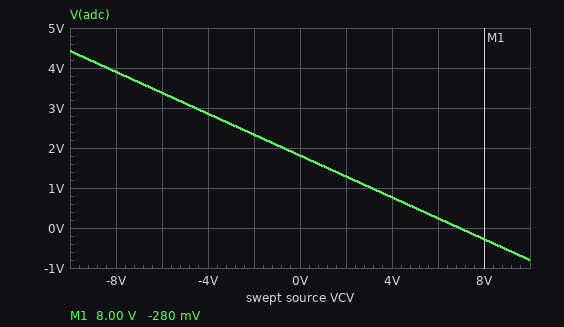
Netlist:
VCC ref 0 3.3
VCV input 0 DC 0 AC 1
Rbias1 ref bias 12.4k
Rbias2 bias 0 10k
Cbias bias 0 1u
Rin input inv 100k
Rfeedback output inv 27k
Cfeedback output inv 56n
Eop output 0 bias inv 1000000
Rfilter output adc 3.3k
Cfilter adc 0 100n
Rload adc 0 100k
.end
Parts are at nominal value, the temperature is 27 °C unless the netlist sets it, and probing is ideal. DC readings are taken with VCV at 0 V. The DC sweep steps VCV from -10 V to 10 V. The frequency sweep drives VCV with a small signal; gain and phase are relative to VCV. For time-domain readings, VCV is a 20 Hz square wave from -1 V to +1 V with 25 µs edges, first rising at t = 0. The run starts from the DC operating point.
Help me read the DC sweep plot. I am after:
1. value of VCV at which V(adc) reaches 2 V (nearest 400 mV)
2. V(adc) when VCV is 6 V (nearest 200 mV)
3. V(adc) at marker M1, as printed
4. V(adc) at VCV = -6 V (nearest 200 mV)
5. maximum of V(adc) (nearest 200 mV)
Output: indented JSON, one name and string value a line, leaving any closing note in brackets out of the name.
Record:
{
  "value of VCV at which V(adc) reaches 2 V": "-800 mV",
  "V(adc) when VCV is 6 V": "200 mV",
  "V(adc) at marker M1, as printed": "-280 mV",
  "V(adc) at VCV = -6 V": "3.4 V",
  "maximum of V(adc)": "4.4 V"
}
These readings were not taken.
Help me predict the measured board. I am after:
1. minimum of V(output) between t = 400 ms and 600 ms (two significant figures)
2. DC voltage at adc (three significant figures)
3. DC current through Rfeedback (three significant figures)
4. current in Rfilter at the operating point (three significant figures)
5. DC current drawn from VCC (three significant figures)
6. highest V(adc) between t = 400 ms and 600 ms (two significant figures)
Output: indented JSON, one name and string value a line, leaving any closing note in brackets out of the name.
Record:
{
  "minimum of V(output) between t = 400 ms and 600 ms": "1.6 V",
  "DC voltage at adc": "1.81 V",
  "DC current through Rfeedback": "14.7 µA",
  "current in Rfilter at the operating point": "18.1 µA",
  "DC current drawn from VCC": "147 µA",
  "highest V(adc) between t = 400 ms and 600 ms": "2.1 V"
}
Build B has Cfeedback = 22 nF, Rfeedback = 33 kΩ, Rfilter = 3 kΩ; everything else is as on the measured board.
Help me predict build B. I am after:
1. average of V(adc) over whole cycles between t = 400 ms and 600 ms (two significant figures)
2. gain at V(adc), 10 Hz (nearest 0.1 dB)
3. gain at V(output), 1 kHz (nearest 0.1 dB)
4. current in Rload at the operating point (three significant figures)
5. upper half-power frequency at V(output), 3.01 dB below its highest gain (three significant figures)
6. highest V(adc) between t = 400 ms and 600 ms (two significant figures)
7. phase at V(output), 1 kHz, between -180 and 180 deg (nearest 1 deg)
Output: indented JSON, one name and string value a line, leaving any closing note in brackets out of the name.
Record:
{
  "average of V(adc) over whole cycles between t = 400 ms and 600 ms": "1.9 V",
  "gain at V(adc), 10 Hz": "-9.9 dB",
  "gain at V(output), 1 kHz": "-23.0 dB",
  "current in Rload at the operating point": "19.0 µA",
  "upper half-power frequency at V(output), 3.01 dB below its highest gain": "219 Hz",
  "highest V(adc) between t = 400 ms and 600 ms": "2.2 V",
  "phase at V(output), 1 kHz, between -180 and 180 deg": "102 deg"
}
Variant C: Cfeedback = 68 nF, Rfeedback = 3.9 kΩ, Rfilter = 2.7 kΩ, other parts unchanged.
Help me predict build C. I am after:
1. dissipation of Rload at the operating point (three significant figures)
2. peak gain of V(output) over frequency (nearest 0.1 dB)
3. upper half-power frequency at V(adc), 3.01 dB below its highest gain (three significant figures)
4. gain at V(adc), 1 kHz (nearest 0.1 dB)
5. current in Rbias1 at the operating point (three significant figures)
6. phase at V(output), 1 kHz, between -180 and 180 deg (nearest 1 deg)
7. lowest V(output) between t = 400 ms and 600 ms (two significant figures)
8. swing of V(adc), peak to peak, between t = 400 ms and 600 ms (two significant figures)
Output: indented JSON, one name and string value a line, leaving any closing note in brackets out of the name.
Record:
{
  "dissipation of Rload at the operating point": "22.2 µW",
  "peak gain of V(output) over frequency": "-28.2 dB",
  "upper half-power frequency at V(adc), 3.01 dB below its highest gain": "388 Hz",
  "gain at V(adc), 1 kHz": "-39.9 dB",
  "current in Rbias1 at the operating point": "147 µA",
  "phase at V(output), 1 kHz, between -180 and 180 deg": "121 deg",
  "lowest V(output) between t = 400 ms and 600 ms": "1.5 V",
  "swing of V(adc), peak to peak, between t = 400 ms and 600 ms": "76 mV"
}
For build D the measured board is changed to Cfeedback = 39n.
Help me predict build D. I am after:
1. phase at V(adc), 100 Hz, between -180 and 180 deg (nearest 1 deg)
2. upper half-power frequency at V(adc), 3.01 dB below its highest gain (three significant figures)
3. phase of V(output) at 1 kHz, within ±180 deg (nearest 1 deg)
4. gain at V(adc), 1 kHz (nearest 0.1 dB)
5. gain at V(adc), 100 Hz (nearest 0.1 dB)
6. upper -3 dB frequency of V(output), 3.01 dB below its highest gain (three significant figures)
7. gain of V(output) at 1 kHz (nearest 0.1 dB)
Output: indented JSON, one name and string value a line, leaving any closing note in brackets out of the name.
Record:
{
  "phase at V(adc), 100 Hz, between -180 and 180 deg": "135 deg",
  "upper half-power frequency at V(adc), 3.01 dB below its highest gain": "140 Hz",
  "phase of V(output) at 1 kHz, within ±180 deg": "99 deg",
  "gain at V(adc), 1 kHz": "-35.2 dB",
  "gain at V(adc), 100 Hz": "-13.4 dB",
  "upper -3 dB frequency of V(output), 3.01 dB below its highest gain": "151 Hz",
  "gain of V(output) at 1 kHz": "-27.9 dB"
}
